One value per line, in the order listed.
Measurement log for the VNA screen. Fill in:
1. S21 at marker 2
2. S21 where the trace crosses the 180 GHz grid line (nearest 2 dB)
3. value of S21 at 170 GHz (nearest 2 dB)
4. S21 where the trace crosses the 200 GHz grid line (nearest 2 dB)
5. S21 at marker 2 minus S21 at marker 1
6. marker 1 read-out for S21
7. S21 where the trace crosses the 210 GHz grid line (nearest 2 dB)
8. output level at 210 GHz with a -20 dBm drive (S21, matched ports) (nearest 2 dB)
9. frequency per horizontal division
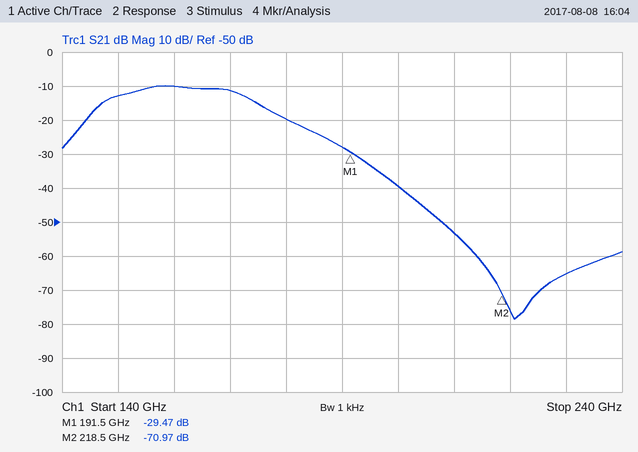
-70.97 dB
-20 dB
-12 dB
-40 dB
-41.50 dB
-29.47 dB
-54 dB
-74 dBm
10 GHz
